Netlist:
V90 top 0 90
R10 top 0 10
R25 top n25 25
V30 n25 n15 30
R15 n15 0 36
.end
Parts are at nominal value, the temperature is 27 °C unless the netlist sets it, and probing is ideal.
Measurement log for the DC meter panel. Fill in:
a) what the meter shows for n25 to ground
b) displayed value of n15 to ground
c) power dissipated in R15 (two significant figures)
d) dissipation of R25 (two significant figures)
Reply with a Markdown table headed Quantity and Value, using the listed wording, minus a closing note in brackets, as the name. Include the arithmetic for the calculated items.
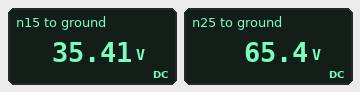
| Quantity | Value |
|---|---|
| what the meter shows for n25 to ground | 65.4 V |
| displayed value of n15 to ground | 35.41 V |
| power dissipated in R15 | (35.41 V)^2 / 36 Ω = 35 W |
| dissipation of R25 | (90 V - 65.4 V)^2 / 25 Ω = 24 W |
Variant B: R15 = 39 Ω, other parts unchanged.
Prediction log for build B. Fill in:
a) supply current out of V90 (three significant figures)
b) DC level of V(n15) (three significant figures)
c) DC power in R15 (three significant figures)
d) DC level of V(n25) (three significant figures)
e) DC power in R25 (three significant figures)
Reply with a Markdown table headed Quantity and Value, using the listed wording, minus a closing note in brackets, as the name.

| Quantity | Value |
|---|---|
| supply current out of V90 | 9.94 A |
| DC level of V(n15) | 36.6 V |
| DC power in R15 | 34.3 W |
| DC level of V(n25) | 66.6 V |
| DC power in R25 | 22.0 W |
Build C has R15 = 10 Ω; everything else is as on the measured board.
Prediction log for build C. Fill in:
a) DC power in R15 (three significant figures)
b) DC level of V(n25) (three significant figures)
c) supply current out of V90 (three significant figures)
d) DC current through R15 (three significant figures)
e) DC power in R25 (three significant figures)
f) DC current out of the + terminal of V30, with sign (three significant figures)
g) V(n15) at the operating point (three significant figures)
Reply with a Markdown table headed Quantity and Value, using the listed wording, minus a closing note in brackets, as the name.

| Quantity | Value |
|---|---|
| DC power in R15 | 29.4 W |
| DC level of V(n25) | 47.1 V |
| supply current out of V90 | 10.7 A |
| DC current through R15 | 1.71 A |
| DC power in R25 | 73.5 W |
| DC current out of the + terminal of V30, with sign | -1.71 A |
| V(n15) at the operating point | 17.1 V |
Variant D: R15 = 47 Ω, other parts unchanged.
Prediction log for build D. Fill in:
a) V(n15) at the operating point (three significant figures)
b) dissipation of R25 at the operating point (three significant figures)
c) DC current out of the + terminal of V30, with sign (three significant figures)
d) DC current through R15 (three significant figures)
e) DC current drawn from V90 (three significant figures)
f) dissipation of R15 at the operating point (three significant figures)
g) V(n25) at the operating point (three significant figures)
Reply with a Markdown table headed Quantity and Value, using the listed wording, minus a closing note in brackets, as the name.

| Quantity | Value |
|---|---|
| V(n15) at the operating point | 39.2 V |
| dissipation of R25 at the operating point | 17.4 W |
| DC current out of the + terminal of V30, with sign | -833 mA |
| DC current through R15 | 833 mA |
| DC current drawn from V90 | 9.83 A |
| dissipation of R15 at the operating point | 32.6 W |
| V(n25) at the operating point | 69.2 V |
